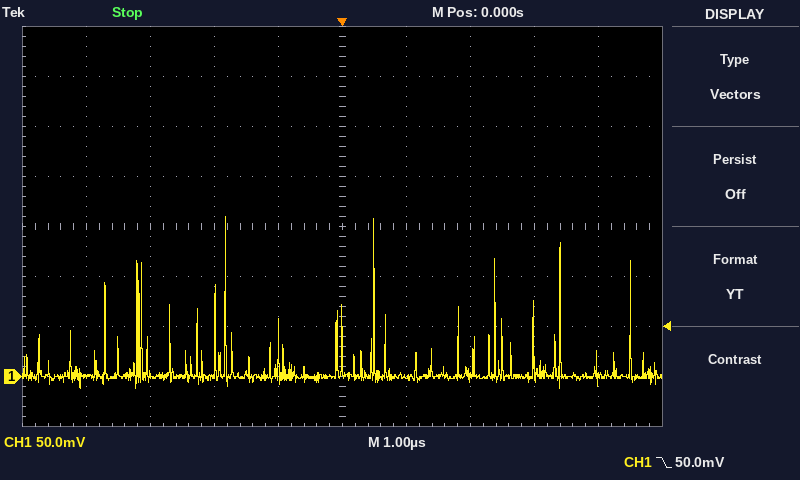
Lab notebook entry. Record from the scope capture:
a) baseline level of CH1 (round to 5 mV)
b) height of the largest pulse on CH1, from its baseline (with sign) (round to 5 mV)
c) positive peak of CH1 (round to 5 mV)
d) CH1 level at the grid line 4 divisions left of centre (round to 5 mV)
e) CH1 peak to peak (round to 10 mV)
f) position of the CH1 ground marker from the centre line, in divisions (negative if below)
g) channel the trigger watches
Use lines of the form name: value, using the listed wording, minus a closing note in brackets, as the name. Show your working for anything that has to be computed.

baseline level of CH1: 0 mV
height of the largest pulse on CH1, from its baseline (with sign): 160 mV − (0 mV) = +160 mV
positive peak of CH1: 160 mV
CH1 level at the grid line 4 divisions left of centre: 0 mV
CH1 peak to peak: 170 mV
position of the CH1 ground marker from the centre line, in divisions: -3.0 div
channel the trigger watches: CH1
